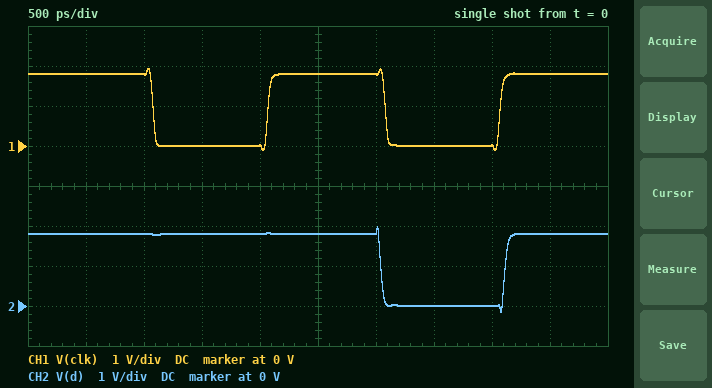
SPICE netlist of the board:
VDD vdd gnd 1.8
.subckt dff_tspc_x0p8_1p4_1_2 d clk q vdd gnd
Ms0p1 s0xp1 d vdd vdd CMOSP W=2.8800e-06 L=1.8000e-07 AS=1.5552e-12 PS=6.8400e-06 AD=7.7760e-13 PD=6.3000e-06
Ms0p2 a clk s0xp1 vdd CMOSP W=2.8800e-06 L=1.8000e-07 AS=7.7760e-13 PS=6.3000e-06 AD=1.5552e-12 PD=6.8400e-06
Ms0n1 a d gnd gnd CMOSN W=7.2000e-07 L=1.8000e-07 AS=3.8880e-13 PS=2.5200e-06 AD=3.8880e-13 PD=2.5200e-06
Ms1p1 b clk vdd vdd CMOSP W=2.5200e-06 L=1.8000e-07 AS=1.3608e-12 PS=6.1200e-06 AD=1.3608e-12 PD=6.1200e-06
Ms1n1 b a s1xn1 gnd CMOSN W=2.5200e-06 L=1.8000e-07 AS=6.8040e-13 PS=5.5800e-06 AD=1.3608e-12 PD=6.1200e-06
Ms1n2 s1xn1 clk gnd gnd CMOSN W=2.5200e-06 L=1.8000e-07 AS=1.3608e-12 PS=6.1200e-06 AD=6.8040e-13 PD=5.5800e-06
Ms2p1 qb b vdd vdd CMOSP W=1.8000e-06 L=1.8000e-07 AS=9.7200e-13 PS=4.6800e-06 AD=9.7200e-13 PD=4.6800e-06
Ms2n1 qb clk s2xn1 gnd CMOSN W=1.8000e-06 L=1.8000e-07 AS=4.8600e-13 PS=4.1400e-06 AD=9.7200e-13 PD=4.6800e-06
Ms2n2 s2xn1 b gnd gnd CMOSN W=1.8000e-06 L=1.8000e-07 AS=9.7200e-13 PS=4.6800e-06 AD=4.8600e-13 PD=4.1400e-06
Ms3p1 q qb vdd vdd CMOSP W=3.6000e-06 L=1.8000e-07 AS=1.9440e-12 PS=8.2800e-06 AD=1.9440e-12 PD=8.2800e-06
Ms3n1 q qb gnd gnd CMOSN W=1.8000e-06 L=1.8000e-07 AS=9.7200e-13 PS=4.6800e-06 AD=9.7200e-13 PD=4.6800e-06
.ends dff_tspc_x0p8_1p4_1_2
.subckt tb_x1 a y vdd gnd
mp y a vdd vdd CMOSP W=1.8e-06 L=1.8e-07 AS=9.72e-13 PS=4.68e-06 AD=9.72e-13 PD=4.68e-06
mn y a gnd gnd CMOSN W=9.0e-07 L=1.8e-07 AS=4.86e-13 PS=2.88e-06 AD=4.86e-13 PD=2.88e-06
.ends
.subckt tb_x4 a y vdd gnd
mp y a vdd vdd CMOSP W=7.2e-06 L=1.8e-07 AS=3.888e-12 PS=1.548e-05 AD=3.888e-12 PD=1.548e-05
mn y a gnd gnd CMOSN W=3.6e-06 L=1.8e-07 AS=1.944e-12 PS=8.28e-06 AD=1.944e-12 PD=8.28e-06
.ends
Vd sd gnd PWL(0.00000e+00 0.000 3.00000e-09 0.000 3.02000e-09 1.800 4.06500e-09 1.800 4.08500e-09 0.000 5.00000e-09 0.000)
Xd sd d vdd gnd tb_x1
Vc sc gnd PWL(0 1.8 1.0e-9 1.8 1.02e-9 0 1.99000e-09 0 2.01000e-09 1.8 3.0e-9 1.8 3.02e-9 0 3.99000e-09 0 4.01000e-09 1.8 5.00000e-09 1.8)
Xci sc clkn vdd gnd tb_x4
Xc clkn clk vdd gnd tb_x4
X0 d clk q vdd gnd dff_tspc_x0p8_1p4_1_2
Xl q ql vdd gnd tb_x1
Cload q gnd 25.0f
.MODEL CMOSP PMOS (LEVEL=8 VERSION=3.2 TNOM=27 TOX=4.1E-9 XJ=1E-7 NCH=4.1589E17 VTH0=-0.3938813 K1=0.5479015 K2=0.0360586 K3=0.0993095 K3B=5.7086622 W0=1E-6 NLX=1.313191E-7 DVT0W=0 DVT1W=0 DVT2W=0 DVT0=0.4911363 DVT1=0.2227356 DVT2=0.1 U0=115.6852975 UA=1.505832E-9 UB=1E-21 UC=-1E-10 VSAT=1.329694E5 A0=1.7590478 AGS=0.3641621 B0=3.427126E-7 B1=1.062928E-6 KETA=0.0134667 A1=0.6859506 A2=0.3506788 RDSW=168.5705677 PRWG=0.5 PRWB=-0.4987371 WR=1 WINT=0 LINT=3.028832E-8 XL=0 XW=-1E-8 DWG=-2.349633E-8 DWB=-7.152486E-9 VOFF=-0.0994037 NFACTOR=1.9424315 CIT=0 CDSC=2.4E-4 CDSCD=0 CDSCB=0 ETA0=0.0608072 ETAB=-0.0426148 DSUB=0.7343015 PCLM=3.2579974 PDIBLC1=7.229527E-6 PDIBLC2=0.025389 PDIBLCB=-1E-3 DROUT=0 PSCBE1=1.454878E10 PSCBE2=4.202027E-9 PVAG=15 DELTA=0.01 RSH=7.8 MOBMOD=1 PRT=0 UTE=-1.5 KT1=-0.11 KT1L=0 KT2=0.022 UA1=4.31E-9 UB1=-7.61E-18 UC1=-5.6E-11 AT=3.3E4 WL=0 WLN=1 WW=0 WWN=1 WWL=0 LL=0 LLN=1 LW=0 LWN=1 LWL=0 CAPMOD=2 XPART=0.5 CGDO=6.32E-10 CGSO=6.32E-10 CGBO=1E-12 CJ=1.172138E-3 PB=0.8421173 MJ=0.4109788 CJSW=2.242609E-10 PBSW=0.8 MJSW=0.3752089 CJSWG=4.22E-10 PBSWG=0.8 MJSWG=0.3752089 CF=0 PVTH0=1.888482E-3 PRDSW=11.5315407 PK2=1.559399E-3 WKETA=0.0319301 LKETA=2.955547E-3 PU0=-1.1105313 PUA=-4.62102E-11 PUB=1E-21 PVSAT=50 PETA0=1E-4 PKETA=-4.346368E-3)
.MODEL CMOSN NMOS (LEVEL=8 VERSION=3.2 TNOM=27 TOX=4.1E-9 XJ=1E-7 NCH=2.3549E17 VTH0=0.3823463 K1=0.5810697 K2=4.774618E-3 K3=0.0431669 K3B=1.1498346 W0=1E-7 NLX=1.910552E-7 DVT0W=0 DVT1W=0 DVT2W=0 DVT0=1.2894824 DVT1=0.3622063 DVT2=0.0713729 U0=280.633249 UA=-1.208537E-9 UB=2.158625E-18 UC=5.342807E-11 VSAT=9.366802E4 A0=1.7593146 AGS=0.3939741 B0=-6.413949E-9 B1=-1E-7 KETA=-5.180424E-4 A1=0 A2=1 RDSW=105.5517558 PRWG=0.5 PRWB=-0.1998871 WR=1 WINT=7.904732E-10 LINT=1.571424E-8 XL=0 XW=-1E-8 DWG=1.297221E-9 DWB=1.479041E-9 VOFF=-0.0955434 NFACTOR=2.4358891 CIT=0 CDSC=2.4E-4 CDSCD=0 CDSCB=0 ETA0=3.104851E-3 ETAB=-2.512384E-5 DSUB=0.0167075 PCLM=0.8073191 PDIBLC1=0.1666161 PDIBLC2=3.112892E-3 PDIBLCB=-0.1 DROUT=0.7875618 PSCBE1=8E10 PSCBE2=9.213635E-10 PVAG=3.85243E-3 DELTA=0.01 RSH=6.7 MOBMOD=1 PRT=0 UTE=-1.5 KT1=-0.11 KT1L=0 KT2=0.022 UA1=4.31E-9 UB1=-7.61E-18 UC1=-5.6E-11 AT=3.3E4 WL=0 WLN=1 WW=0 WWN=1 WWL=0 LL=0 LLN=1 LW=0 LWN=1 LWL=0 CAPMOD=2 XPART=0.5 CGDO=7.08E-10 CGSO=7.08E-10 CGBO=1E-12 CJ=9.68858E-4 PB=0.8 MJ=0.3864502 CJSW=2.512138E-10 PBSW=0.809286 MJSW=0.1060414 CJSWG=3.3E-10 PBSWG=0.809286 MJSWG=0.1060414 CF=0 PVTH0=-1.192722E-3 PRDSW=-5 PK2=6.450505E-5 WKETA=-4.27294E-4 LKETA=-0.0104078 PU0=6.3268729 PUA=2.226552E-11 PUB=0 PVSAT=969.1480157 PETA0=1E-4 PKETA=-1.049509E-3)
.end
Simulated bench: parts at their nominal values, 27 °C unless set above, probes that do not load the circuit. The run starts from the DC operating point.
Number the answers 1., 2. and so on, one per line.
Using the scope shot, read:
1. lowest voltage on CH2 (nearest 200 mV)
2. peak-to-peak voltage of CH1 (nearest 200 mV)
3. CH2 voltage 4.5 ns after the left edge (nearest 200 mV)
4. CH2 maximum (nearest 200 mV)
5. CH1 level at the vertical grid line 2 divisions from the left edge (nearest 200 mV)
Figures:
1. -200 mV
2. 2.0 V
3. 1.8 V
4. 2.0 V
5. 1.8 V
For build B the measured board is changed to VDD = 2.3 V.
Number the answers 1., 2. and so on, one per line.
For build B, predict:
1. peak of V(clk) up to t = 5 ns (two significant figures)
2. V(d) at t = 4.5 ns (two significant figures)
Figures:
1. 2.4 V
2. 2.3 V
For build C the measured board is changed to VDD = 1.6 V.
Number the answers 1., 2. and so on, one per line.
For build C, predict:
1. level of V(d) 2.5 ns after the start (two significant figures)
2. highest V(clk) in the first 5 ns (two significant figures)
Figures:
1. 1.6 V
2. 1.7 V
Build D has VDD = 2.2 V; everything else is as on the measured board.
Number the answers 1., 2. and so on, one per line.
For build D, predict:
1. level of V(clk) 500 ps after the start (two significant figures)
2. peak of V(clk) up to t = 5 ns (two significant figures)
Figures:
1. 2.2 V
2. 2.3 V
